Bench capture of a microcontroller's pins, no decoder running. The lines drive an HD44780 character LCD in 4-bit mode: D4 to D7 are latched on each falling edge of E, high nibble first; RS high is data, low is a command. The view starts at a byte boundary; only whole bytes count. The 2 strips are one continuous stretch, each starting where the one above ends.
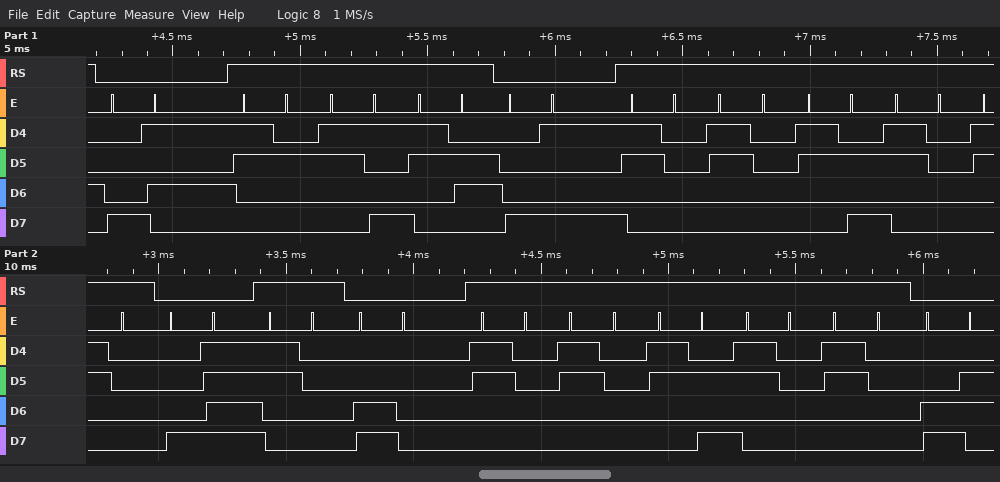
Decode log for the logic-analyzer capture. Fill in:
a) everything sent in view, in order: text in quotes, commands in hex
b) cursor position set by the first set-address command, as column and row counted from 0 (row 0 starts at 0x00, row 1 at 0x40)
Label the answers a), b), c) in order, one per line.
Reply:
a) 0x85 "296" 0x89 "00:00" 0x8F "0" 0xC0 "00:00" 0xC6
b) column 5, row 0
